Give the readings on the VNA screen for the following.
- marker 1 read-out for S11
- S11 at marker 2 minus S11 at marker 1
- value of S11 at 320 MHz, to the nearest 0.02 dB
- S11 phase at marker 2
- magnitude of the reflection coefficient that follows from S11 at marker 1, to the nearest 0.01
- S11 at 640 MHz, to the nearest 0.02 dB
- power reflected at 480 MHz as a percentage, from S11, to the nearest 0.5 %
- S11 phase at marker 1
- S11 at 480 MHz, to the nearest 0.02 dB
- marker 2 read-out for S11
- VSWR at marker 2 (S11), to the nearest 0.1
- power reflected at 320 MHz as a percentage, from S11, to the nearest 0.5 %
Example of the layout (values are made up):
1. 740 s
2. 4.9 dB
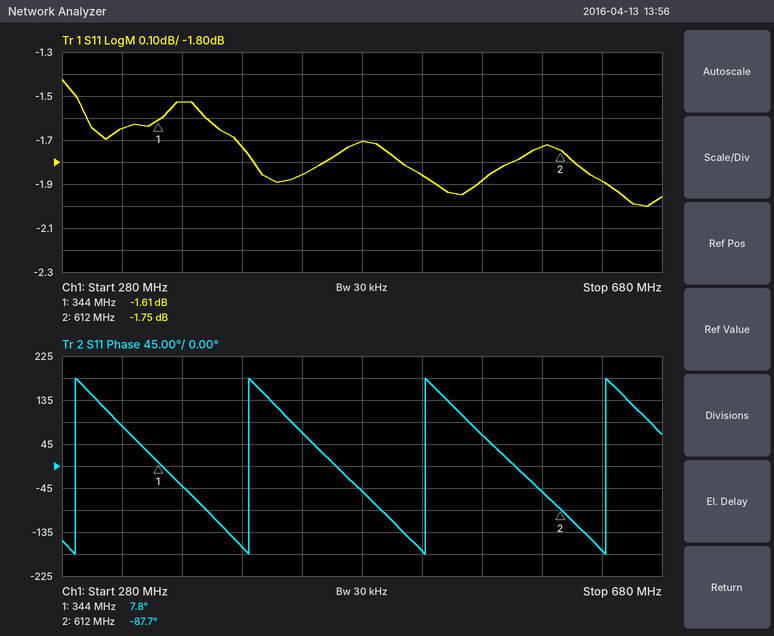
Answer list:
1. -1.61 dB
2. -0.14 dB
3. -1.64 dB
4. -87.7°
5. 0.83
6. -1.88 dB
7. 67.5 %
8. 7.8°
9. -1.70 dB
10. -1.75 dB
11. 10.0
12. 68.5 %
